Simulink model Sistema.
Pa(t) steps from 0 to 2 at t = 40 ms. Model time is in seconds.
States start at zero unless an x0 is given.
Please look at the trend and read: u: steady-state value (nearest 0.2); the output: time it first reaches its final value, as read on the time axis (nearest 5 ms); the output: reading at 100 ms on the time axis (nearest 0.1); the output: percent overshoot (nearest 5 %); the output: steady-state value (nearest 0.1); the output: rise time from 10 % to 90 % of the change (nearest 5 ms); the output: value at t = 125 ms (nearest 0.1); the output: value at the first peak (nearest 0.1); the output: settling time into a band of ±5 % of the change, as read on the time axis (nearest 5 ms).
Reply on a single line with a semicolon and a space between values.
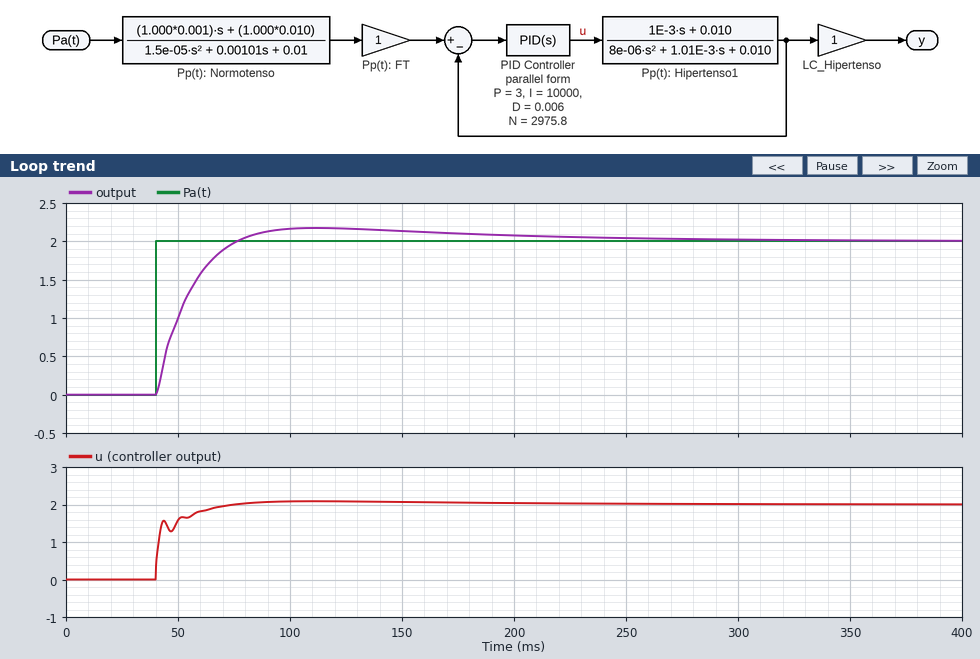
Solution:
2.0; 75 ms; 2.2; 10 %; 2.0; 25 ms; 2.2; 2.2; 175 ms
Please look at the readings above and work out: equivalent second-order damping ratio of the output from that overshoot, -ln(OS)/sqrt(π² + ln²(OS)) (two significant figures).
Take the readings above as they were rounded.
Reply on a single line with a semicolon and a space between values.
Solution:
0.59
